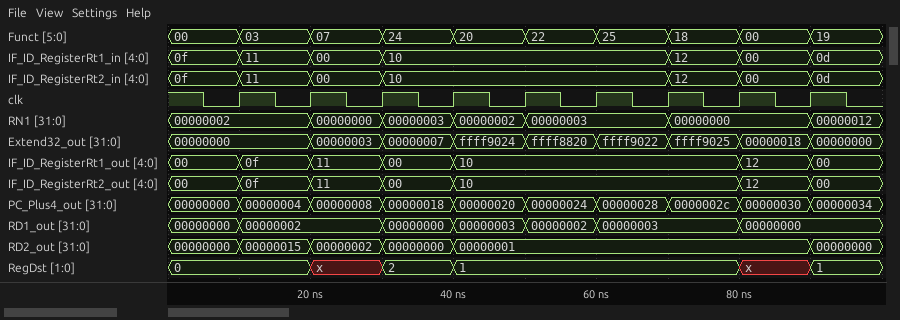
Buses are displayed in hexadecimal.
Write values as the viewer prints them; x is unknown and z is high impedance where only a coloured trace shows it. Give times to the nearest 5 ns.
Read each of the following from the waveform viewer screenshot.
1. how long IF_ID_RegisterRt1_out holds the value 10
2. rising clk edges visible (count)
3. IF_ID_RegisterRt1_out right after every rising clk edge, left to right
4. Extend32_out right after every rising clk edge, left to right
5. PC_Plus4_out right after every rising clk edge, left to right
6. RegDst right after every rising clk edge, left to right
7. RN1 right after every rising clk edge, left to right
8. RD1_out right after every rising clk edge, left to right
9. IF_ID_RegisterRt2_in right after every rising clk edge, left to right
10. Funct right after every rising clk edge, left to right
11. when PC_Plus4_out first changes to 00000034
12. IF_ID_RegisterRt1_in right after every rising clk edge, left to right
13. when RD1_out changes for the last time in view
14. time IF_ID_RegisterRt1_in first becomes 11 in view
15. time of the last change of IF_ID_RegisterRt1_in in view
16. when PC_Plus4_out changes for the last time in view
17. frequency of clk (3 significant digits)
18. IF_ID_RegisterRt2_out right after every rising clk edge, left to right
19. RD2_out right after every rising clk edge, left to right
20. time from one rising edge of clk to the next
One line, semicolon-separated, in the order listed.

40 ns; 9; 0f, 11, 00, 10, 10, 10, 10, 12, 00; 00000000, 00000003, 00000007, ffff9024, ffff8820, ffff9022, ffff9025, 00000018, 00000000; 00000004, 00000008, 00000018, 00000020, 00000024, 00000028, 0000002c, 00000030, 00000034; 0, x, 2, 1, 1, 1, 1, x, 1; 00000002, 00000000, 00000003, 00000002, 00000003, 00000003, 00000000, 00000000, 00000012; 00000002, 00000002, 00000000, 00000003, 00000002, 00000003, 00000003, 00000000, 00000000; 11, 00, 10, 10, 10, 10, 12, 00, 0d; 03, 07, 24, 20, 22, 25, 18, 00, 19; 90 ns; 11, 00, 10, 10, 10, 10, 12, 00, 0d; 80 ns; 10 ns; 90 ns; 90 ns; 100 MHz; 0f, 11, 00, 10, 10, 10, 10, 12, 00; 00000015, 00000002, 00000000, 00000001, 00000001, 00000001, 00000001, 00000001, 00000000; 10 ns
